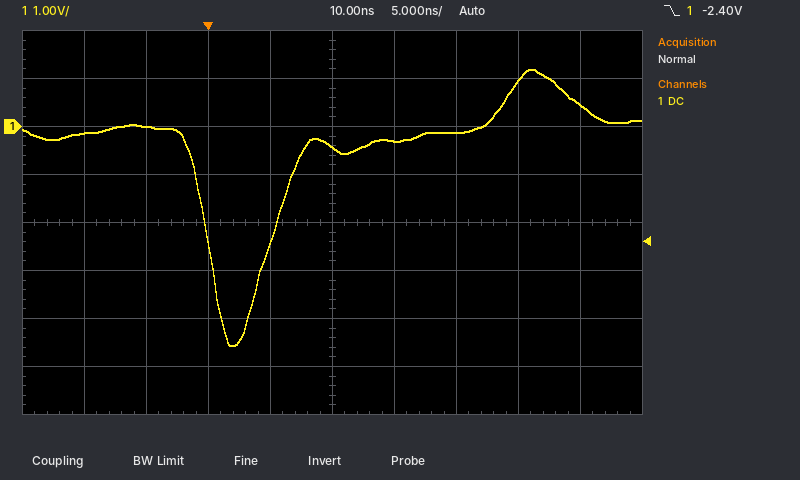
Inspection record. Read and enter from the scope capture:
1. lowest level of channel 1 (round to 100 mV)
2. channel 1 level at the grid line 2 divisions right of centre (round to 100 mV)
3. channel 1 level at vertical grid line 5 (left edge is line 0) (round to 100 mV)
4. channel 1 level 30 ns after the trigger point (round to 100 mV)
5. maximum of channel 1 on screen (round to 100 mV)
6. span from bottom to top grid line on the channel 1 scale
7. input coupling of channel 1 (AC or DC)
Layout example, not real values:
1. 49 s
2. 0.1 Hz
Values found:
1. -4.6 V
2. -100 mV
3. -400 mV
4. 500 mV
5. 1.2 V
6. 8 V
7. DC
